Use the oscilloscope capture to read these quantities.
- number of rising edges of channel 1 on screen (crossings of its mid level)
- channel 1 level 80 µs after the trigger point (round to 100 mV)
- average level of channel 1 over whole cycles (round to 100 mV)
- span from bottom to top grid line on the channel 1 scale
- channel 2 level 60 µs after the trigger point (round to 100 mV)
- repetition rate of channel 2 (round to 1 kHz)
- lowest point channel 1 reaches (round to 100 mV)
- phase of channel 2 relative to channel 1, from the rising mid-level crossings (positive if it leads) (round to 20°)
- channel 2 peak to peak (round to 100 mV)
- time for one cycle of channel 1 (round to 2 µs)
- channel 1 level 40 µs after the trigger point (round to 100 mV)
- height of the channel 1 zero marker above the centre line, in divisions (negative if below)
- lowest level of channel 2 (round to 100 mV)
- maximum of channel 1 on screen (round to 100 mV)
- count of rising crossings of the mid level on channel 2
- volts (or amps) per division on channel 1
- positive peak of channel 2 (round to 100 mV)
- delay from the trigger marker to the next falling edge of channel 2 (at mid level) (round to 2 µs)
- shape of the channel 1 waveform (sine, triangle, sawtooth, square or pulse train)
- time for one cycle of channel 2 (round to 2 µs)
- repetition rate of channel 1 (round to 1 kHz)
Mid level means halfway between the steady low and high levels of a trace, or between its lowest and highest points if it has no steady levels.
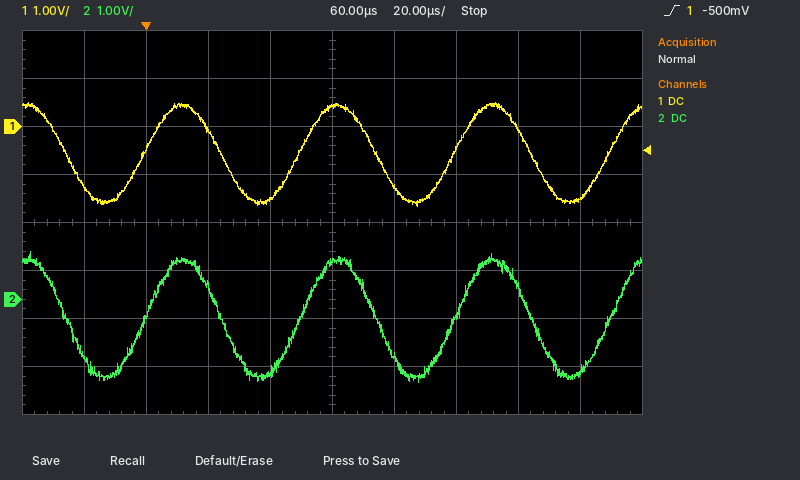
4
-1.2 V
-600 mV
8 V
800 mV
20 kHz
-1.7 V
0°
2.7 V
50 µs
-1.5 V
+2.0 div
-1.7 V
500 mV
4
1 V
1.0 V
24 µs
sine
50 µs
20 kHz
